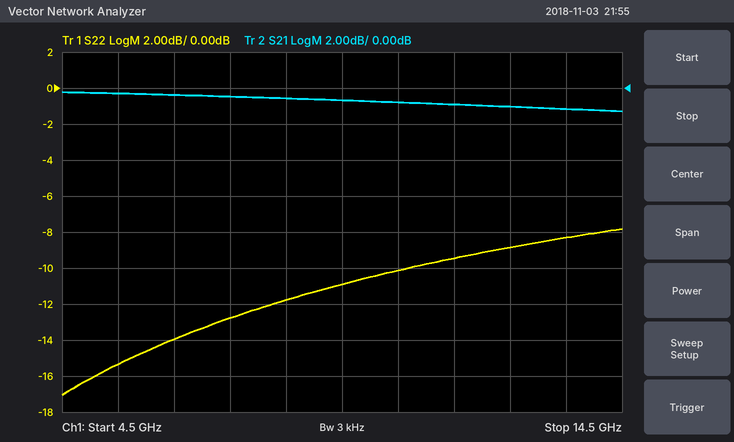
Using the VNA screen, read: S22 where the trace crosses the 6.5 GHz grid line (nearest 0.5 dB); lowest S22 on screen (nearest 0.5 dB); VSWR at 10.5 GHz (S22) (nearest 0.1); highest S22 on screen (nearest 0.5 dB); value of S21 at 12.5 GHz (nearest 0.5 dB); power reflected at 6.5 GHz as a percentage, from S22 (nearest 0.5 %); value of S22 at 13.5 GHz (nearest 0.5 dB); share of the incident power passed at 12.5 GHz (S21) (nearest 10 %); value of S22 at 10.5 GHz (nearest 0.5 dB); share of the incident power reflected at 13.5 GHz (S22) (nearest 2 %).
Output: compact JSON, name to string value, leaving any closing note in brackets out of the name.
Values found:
{"S22 where the trace crosses the 6.5 GHz grid line": "-14.0 dB", "lowest S22 on screen": "-17.0 dB", "VSWR at 10.5 GHz (S22)": "1.9", "highest S22 on screen": "-8.0 dB", "value of S21 at 12.5 GHz": "-1.0 dB", "power reflected at 6.5 GHz as a percentage, from S22": "4.0 %", "value of S22 at 13.5 GHz": "-8.5 dB", "share of the incident power passed at 12.5 GHz (S21)": "80 %", "value of S22 at 10.5 GHz": "-10.0 dB", "share of the incident power reflected at 13.5 GHz (S22)": "14 %"}
